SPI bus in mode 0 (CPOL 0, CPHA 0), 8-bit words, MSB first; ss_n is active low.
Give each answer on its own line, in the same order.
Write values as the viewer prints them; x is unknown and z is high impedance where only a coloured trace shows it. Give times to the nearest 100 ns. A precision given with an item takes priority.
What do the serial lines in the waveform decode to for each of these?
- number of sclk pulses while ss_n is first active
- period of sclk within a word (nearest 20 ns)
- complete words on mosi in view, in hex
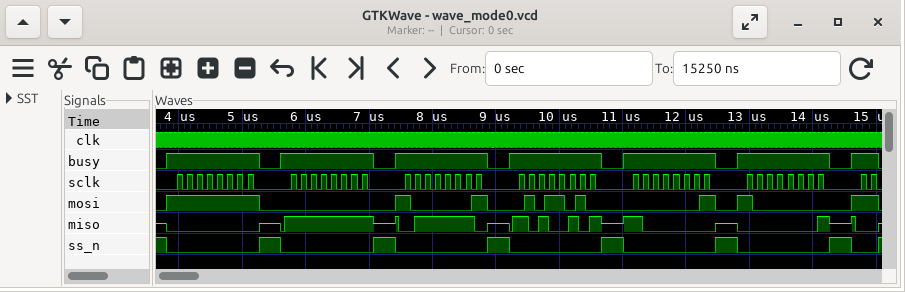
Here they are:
8
160 ns
FF, 00, 81, 5A, 01, 80
